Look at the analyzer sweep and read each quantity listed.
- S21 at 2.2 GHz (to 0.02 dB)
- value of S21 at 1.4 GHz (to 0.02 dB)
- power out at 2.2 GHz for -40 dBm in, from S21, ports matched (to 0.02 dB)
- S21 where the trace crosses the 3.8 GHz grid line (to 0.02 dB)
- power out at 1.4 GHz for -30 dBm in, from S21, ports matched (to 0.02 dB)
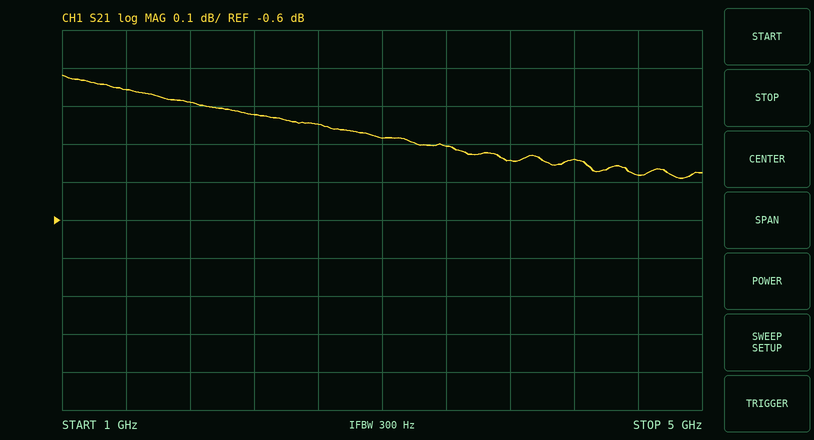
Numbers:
-0.32 dB
-0.26 dB
-40.32 dBm
-0.44 dB
-30.26 dBm
